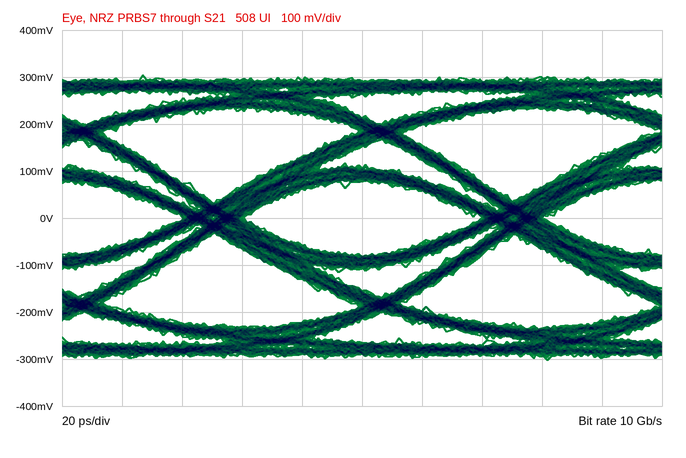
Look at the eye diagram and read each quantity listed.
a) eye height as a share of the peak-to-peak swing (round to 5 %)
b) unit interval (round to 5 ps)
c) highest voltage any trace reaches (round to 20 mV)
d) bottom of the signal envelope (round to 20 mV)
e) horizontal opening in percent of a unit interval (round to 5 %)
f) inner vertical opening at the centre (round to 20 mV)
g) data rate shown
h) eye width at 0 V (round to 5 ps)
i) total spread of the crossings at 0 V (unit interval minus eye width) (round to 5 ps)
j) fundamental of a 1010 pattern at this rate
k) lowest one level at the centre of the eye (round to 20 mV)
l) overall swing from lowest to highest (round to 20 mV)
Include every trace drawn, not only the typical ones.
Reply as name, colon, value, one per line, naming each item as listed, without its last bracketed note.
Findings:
eye height as a share of the peak-to-peak swing: 25 %
unit interval: 100 ps
highest voltage any trace reaches: 300 mV
bottom of the signal envelope: -300 mV
horizontal opening in percent of a unit interval: 80 %
inner vertical opening at the centre: 160 mV
data rate shown: 10 Gb/s
eye width at 0 V: 80 ps
total spread of the crossings at 0 V (unit interval minus eye width): 20 ps
fundamental of a 1010 pattern at this rate: 5 GHz
lowest one level at the centre of the eye: 80 mV
overall swing from lowest to highest: 600 mV
